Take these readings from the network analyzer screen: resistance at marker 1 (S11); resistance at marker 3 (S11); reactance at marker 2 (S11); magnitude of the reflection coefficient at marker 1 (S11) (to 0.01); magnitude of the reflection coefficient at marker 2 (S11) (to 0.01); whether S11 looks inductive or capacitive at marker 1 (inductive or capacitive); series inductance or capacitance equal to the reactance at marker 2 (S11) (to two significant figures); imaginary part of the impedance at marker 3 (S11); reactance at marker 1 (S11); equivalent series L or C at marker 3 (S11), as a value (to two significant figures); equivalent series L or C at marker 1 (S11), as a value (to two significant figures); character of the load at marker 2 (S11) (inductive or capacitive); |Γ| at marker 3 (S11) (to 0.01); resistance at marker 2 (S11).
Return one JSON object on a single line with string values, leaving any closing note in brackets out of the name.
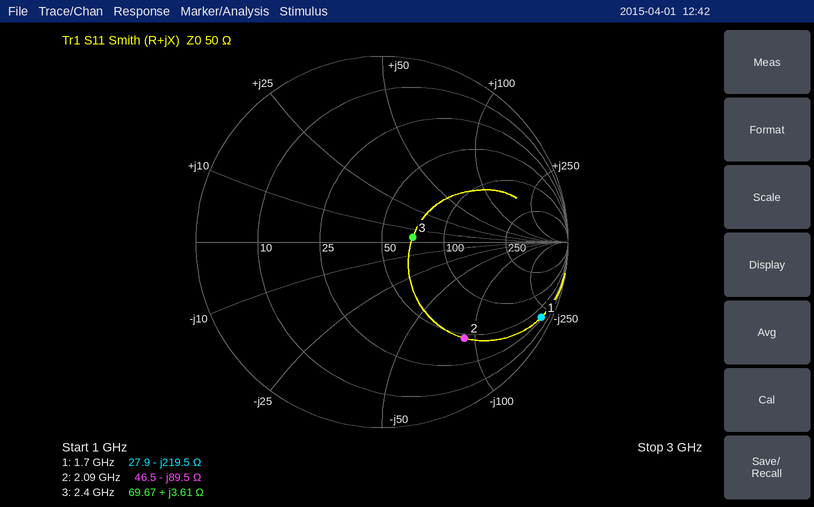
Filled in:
{"resistance at marker 1": "27.9 Ω", "resistance at marker 3": "69.67 Ω", "reactance at marker 2": "-89.5 Ω", "magnitude of the reflection coefficient at marker 1 (S11)": "0.95", "magnitude of the reflection coefficient at marker 2 (S11)": "0.68", "whether S11 looks inductive or capacitive at marker 1": "capacitive", "series inductance or capacitance equal to the reactance at marker 2 (S11)": "850 fF", "imaginary part of the impedance at marker 3": "+3.61 Ω", "reactance at marker 1": "-219.5 Ω", "equivalent series L or C at marker 3 (S11), as a value": "240 pH", "equivalent series L or C at marker 1 (S11), as a value": "430 fF", "character of the load at marker 2 (S11)": "capacitive", "|Γ| at marker 3 (S11)": "0.17", "resistance at marker 2": "46.5 Ω"}
